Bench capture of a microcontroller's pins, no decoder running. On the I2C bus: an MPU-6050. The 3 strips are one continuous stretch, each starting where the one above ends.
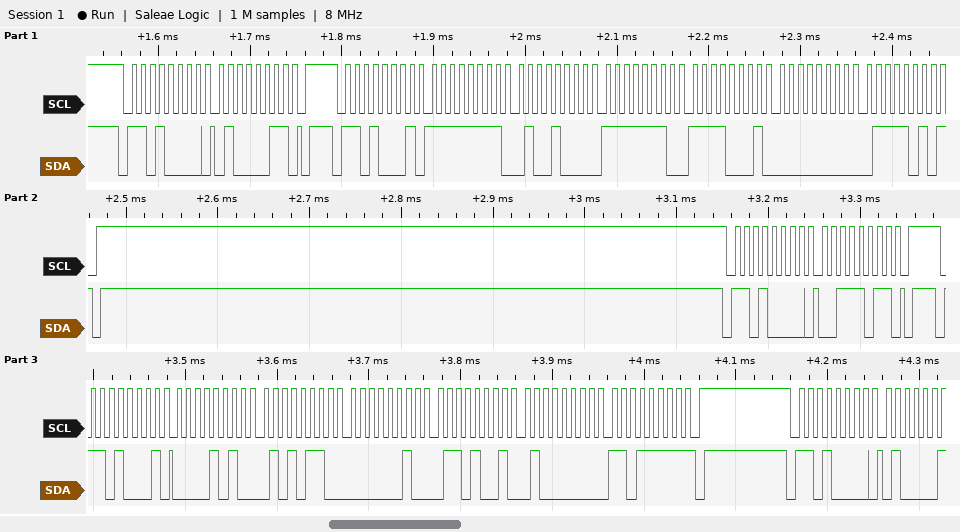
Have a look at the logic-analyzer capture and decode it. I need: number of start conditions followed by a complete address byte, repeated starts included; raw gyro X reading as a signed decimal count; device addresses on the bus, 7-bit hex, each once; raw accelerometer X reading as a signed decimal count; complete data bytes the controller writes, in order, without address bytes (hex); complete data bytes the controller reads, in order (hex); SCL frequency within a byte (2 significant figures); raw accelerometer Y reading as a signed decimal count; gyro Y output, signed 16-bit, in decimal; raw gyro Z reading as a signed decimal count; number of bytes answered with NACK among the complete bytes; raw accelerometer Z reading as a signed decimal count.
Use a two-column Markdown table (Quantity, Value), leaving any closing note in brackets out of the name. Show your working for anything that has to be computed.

| Quantity | Value |
|---|---|
| number of start conditions followed by a complete address byte, repeated starts included | 5 |
| raw gyro X reading as a signed decimal count | 0xFF48 = -184 |
| device addresses on the bus, 7-bit hex, each once | 0x68 |
| raw accelerometer X reading as a signed decimal count | 0x0A56 = 2646 |
| complete data bytes the controller writes, in order, without address bytes | 43 3B |
| complete data bytes the controller reads, in order | FF 48 FE F1 00 7A 0A 56 02 69 40 DF |
| SCL frequency within a byte | 100 kHz |
| raw accelerometer Y reading as a signed decimal count | 0x0269 = 617 |
| gyro Y output, signed 16-bit, in decimal | 0xFEF1 = -271 |
| raw gyro Z reading as a signed decimal count | 0x007A = 122 |
| number of bytes answered with NACK among the complete bytes | 2 |
| raw accelerometer Z reading as a signed decimal count | 0x40DF = 16607 |
